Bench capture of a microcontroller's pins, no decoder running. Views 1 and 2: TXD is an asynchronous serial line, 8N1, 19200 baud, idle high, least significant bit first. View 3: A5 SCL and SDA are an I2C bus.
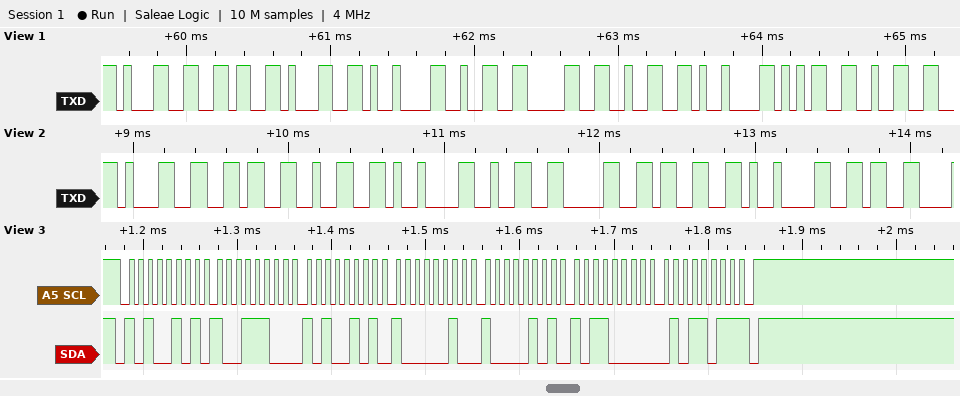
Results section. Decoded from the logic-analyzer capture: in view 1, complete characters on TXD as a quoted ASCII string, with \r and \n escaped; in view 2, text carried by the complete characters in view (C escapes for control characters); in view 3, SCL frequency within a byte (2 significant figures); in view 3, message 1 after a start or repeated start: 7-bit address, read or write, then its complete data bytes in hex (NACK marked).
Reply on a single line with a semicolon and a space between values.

"161\t202\t52"; "162\t203\t6"; 100 kHz; 0x52 read: 9C A5 82 85 B0 5B NACK
